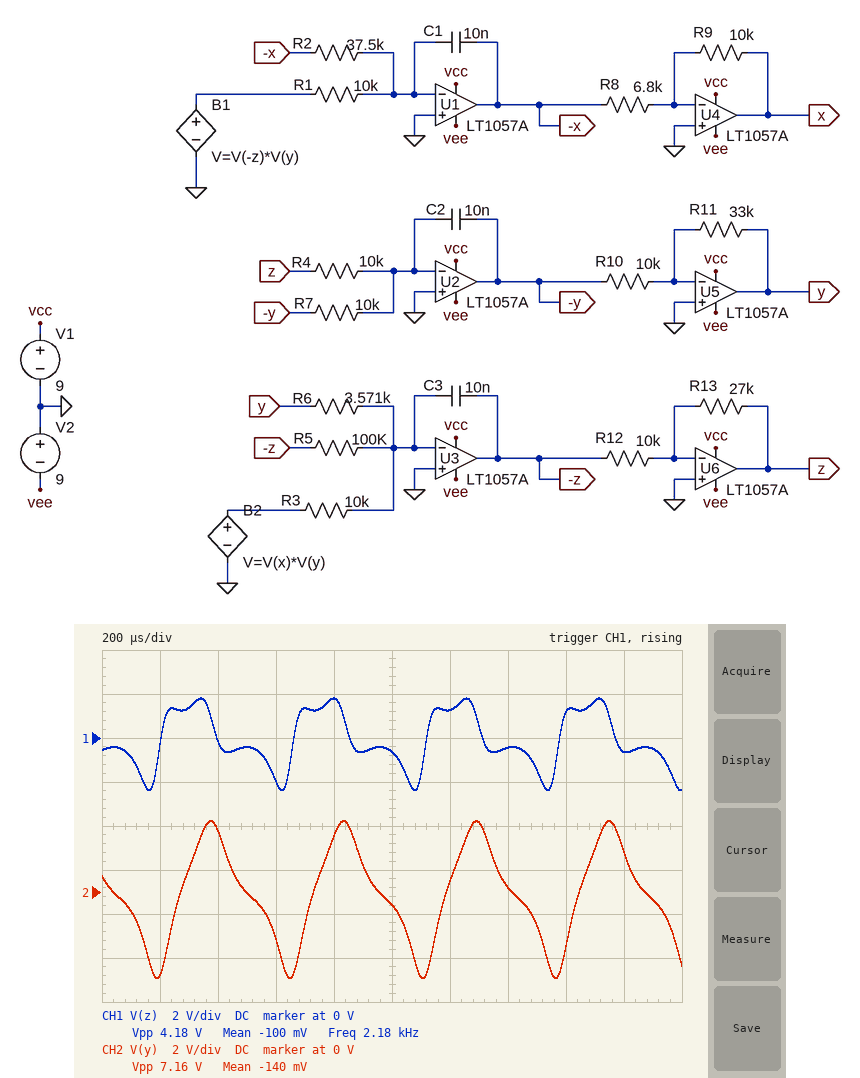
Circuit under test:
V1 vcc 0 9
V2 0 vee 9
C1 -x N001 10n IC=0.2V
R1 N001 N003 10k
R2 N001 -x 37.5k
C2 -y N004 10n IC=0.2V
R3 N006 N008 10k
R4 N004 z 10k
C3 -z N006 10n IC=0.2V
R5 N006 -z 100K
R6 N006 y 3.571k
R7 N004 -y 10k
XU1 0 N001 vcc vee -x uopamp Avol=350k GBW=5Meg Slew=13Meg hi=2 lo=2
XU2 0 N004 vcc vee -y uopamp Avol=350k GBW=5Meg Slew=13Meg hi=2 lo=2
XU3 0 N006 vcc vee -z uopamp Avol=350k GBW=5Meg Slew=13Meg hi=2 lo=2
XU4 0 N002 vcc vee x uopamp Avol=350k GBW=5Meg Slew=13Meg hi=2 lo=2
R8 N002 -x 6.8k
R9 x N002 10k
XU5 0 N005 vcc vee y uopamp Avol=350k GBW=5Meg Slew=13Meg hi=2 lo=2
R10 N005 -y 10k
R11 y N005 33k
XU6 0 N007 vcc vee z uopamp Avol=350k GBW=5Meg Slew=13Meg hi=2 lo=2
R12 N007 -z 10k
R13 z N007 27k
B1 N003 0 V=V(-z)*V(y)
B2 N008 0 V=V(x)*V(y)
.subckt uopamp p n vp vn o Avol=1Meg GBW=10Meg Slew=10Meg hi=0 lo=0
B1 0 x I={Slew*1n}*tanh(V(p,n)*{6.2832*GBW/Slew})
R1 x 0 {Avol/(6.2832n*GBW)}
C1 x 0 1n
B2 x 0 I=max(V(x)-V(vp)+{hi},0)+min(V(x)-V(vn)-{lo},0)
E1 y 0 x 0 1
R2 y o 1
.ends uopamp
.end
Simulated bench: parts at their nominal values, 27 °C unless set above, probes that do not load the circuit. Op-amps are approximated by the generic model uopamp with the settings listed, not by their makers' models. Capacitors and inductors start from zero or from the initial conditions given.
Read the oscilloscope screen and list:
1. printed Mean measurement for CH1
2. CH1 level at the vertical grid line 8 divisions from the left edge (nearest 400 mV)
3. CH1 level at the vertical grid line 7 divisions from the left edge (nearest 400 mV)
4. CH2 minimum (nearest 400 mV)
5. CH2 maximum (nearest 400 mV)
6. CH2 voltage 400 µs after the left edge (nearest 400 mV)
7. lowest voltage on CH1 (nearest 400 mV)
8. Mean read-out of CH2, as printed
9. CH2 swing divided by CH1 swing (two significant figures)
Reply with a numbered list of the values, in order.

1. -100 mV
2. 1.2 V
3. -400 mV
4. -4.0 V
5. 3.2 V
6. 2.8 V
7. -2.4 V
8. -140 mV
9. 1.7
